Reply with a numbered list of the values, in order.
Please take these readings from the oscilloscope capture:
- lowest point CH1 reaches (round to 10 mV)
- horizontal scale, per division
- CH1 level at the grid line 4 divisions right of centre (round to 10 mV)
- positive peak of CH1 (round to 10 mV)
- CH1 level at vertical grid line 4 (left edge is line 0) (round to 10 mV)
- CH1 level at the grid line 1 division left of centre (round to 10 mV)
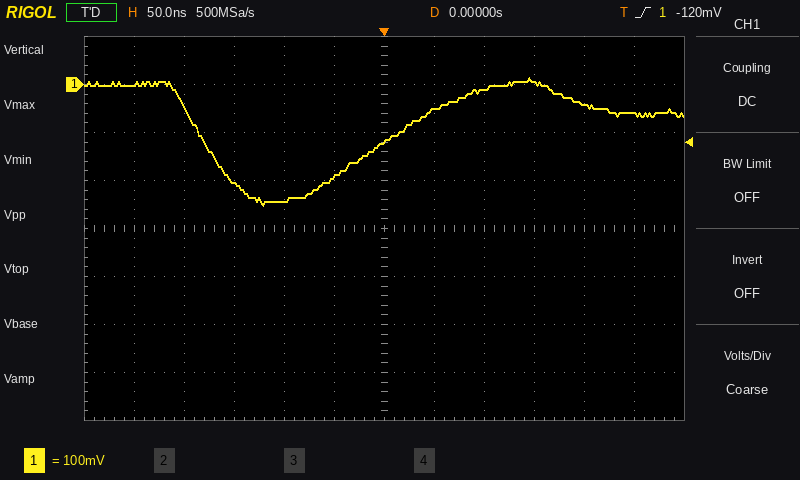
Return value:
1. -250 mV
2. 50 ns
3. -40 mV
4. 10 mV
5. -240 mV
6. -190 mV
